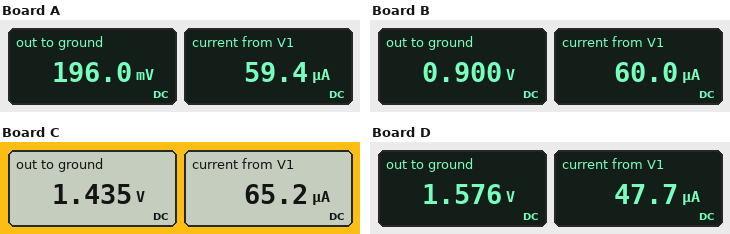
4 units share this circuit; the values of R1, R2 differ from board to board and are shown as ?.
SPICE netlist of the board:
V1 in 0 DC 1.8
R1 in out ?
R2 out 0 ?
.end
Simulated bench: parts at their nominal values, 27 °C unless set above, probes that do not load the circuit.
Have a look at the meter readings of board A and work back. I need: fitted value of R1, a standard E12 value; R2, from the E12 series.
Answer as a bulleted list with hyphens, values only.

- 27 kΩ
- 3.3 kΩ
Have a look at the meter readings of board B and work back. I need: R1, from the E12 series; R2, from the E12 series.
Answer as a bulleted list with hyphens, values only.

- 15 kΩ
- 15 kΩ
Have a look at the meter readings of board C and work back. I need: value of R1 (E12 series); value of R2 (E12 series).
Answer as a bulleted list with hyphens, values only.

- 5.6 kΩ
- 22 kΩ
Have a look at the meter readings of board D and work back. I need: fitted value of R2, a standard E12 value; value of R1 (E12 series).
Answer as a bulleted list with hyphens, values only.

- 33 kΩ
- 4.7 kΩ
